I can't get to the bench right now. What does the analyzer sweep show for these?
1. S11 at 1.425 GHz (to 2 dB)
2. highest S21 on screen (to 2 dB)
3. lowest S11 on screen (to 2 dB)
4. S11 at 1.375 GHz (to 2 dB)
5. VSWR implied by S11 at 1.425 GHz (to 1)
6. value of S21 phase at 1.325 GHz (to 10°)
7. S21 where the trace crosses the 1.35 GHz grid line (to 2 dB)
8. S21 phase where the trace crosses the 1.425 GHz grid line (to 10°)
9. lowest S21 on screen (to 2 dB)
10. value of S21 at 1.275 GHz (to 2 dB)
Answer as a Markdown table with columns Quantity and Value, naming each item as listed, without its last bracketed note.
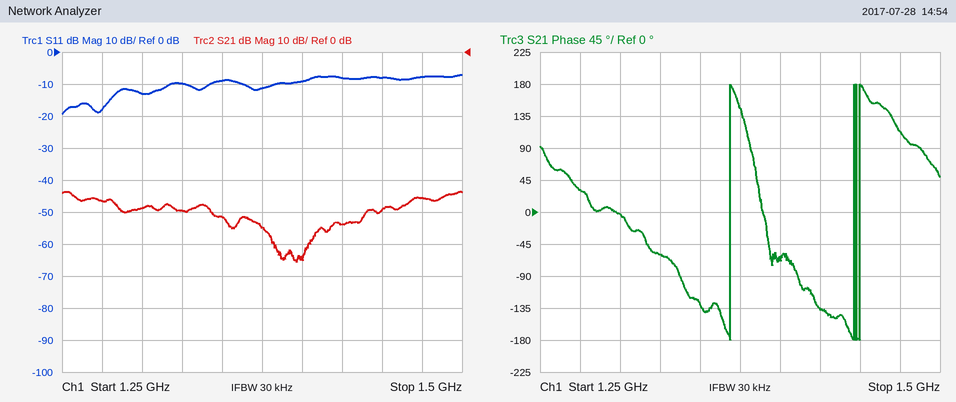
| Quantity | Value |
|---|---|
| S11 at 1.425 GHz | -8 dB |
| highest S21 on screen | -44 dB |
| lowest S11 on screen | -20 dB |
| S11 at 1.375 GHz | -12 dB |
| VSWR implied by S11 at 1.425 GHz | 2 |
| value of S21 phase at 1.325 GHz | -60° |
| S21 where the trace crosses the 1.35 GHz grid line | -52 dB |
| S21 phase where the trace crosses the 1.425 GHz grid line | -140° |
| lowest S21 on screen | -66 dB |
| value of S21 at 1.275 GHz | -46 dB |
